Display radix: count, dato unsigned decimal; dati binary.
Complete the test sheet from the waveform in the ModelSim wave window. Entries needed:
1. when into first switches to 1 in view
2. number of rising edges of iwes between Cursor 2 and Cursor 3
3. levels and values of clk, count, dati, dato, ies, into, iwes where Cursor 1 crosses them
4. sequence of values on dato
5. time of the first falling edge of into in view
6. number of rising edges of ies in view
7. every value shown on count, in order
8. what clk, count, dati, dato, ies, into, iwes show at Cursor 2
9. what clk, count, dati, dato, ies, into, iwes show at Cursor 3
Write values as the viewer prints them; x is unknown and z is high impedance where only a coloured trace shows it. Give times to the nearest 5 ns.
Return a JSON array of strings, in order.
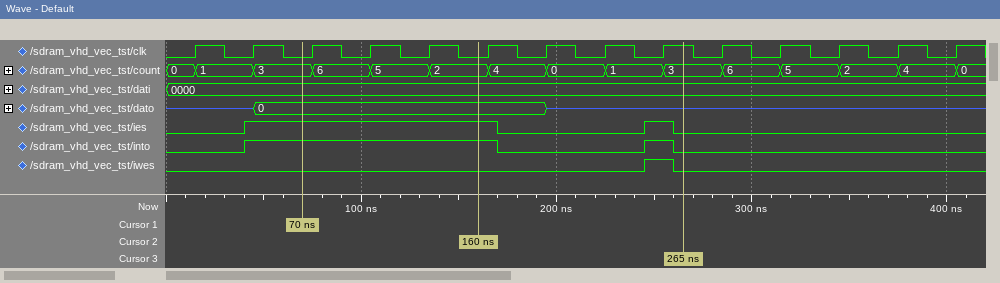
["40 ns", "1", "clk=0, count=3, dati=0000, dato=0, ies=1, into=1, iwes=0", "z, 0, z", "170 ns", "2", "0, 1, 3, 6, 5, 2, 4, 0, 1, 3, 6, 5, 2, 4, 0", "clk=0, count=2, dati=0000, dato=0, ies=1, into=1, iwes=0", "clk=1, count=3, dati=0000, dato=z, ies=0, into=0, iwes=0"]
